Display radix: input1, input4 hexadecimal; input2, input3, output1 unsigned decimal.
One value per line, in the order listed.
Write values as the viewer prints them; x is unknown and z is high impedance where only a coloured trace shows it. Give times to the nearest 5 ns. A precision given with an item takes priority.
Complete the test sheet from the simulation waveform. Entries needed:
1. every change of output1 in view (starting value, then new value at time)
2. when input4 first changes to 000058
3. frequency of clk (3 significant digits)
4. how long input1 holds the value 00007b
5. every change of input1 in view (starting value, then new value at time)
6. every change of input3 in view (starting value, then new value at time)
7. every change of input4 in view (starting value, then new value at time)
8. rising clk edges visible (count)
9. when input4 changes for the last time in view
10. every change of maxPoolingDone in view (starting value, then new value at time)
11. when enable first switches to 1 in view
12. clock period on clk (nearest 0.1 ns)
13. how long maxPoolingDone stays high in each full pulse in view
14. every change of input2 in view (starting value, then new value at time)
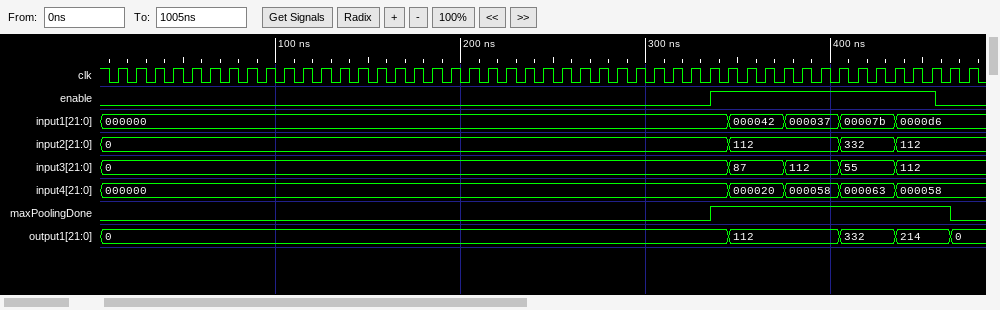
0, 112 at 345 ns, 332 at 405 ns, 214 at 435 ns, 0 at 465 ns
375 ns
100 MHz
30 ns
000000, 000042 at 345 ns, 000037 at 375 ns, 00007b at 405 ns, 0000d6 at 435 ns
0, 87 at 345 ns, 112 at 375 ns, 55 at 405 ns, 112 at 435 ns
000000, 000020 at 345 ns, 000058 at 375 ns, 000063 at 405 ns, 000058 at 435 ns
47
435 ns
0, 1 at 335 ns, 0 at 465 ns
335 ns
10 ns
130 ns
0, 112 at 345 ns, 332 at 405 ns, 112 at 435 ns
